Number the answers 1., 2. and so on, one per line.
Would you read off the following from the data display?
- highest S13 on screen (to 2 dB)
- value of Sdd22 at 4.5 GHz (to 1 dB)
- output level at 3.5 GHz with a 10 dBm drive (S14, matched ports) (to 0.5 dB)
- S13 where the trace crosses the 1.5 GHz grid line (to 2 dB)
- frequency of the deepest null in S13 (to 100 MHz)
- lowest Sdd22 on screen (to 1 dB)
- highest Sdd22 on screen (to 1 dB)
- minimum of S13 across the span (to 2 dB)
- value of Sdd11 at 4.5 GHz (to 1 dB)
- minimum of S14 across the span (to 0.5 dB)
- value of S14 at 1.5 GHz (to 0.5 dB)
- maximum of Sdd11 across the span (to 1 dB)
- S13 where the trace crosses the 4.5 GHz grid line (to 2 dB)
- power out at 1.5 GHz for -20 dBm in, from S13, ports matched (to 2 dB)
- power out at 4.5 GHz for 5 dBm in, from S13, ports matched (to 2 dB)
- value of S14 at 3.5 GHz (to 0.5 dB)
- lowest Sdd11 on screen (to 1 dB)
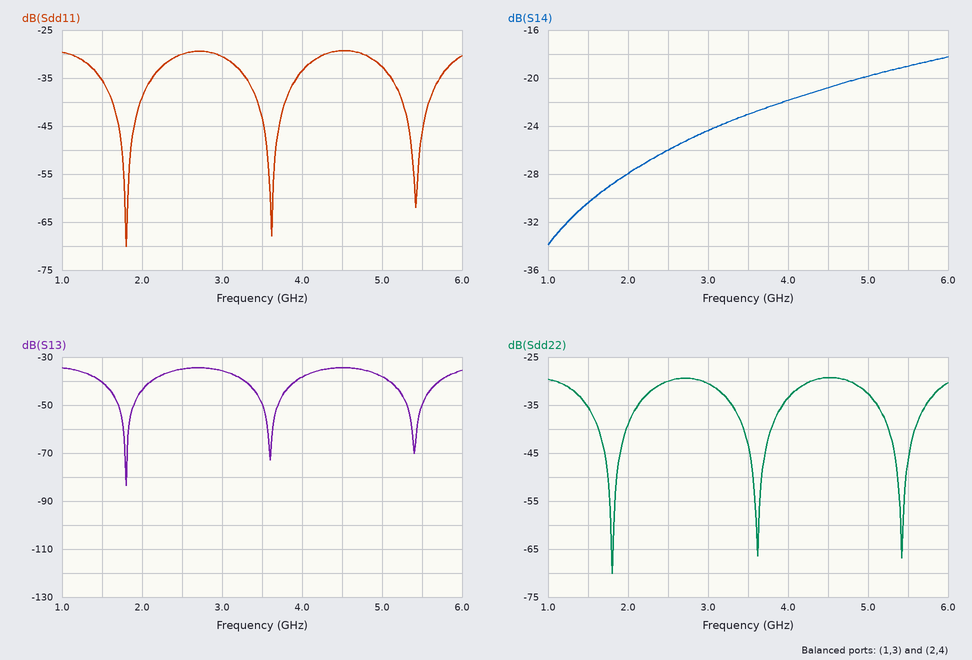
1. -34 dB
2. -29 dB
3. -13.0 dBm
4. -40 dB
5. 1.8 GHz
6. -70 dB
7. -29 dB
8. -84 dB
9. -29 dB
10. -34.0 dB
11. -30.5 dB
12. -29 dB
13. -34 dB
14. -60 dBm
15. -30 dBm
16. -23.0 dB
17. -70 dB
